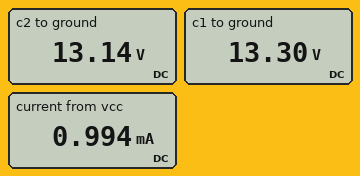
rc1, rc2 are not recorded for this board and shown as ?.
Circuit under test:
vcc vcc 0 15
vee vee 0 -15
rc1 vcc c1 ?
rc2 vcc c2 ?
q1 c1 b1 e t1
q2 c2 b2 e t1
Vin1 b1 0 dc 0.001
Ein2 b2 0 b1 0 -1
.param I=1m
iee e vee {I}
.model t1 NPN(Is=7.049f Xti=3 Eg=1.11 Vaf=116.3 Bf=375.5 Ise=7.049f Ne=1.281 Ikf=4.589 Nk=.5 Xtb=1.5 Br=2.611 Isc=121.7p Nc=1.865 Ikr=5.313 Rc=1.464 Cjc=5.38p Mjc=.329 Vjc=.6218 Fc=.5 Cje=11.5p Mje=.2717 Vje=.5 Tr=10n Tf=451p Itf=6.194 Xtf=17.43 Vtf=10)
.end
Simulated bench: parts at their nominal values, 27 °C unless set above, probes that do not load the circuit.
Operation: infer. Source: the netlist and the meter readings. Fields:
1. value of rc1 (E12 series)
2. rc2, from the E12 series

3.3 kΩ
3.9 kΩ
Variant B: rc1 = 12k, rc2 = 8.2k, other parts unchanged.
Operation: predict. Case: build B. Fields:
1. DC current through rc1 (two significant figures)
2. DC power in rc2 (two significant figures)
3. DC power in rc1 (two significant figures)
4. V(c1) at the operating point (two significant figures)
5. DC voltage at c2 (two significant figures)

510 µA
1.9 mW
3.1 mW
8.9 V
11 V
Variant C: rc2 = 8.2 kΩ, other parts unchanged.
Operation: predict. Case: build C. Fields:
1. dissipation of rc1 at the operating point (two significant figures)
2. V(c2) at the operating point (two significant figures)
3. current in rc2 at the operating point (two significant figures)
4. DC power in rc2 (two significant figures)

890 µW
11 V
470 µA
1.8 mW
